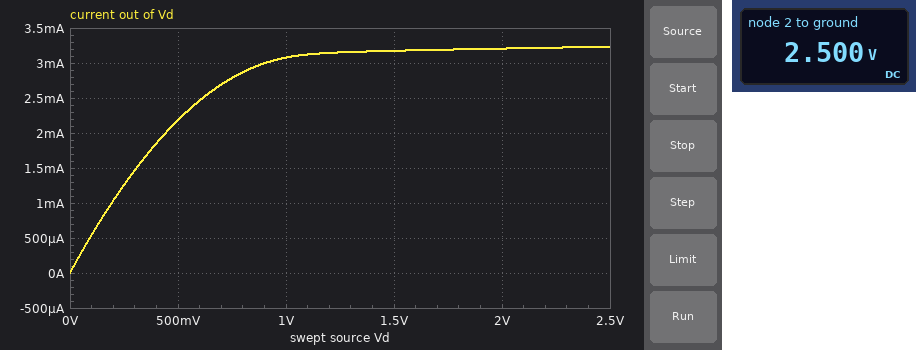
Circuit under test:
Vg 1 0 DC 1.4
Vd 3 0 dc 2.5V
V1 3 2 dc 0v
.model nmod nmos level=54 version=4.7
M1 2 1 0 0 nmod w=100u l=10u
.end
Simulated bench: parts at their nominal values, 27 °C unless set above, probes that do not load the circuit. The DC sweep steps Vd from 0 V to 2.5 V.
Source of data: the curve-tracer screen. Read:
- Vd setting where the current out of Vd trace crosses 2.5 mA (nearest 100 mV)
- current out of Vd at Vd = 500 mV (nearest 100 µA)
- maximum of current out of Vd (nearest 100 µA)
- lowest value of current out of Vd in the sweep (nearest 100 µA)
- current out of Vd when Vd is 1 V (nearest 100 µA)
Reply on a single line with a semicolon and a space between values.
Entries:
600 mV; 2.2 mA; 3.2 mA; 0 A; 3.1 mA
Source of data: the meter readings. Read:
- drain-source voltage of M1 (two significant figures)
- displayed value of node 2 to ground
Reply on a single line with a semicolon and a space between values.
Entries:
2.5 V; 2.500 V
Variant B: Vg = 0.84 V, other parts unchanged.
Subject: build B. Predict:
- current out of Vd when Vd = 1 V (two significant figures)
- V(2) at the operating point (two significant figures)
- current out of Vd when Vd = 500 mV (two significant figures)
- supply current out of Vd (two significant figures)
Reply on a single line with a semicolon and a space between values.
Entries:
1.1 mA; 2.5 V; 1.0 mA; 1.2 mA
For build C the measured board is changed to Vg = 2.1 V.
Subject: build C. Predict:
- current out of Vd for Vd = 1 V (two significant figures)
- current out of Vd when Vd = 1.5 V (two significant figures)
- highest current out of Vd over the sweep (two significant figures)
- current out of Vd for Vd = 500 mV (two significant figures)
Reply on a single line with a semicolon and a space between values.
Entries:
5.4 mA; 6.4 mA; 6.6 mA; 3.3 mA
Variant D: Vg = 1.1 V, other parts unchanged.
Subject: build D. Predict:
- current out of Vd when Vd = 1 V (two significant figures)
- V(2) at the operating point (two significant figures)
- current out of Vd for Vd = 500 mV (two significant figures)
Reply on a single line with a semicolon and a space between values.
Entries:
2.0 mA; 2.5 V; 1.6 mA
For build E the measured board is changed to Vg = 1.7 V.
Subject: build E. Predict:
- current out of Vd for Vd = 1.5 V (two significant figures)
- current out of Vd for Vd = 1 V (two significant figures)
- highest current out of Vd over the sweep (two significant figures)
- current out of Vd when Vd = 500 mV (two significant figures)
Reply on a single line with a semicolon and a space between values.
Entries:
4.5 mA; 4.1 mA; 4.6 mA; 2.7 mA
